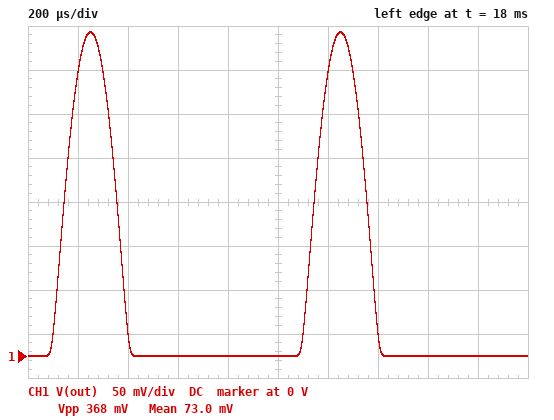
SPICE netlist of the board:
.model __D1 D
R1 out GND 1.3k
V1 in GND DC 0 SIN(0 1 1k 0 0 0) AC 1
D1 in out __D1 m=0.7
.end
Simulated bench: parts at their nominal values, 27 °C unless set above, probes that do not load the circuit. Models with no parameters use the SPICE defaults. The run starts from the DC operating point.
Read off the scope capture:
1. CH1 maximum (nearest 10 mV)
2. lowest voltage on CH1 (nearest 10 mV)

370 mV
0 V
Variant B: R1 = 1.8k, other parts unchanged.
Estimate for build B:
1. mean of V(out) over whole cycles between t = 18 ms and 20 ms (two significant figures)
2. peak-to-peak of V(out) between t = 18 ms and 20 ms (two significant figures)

75 mV
380 mV
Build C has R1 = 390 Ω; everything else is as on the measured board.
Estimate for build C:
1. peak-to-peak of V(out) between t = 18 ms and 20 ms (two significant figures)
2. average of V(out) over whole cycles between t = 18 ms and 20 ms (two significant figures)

340 mV
65 mV
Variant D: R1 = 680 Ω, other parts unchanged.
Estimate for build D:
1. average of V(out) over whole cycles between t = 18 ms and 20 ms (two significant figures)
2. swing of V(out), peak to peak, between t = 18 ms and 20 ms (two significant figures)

68 mV
350 mV
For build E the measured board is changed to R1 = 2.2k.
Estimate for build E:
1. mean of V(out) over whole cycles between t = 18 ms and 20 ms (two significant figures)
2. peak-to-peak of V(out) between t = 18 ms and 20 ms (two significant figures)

77 mV
380 mV
